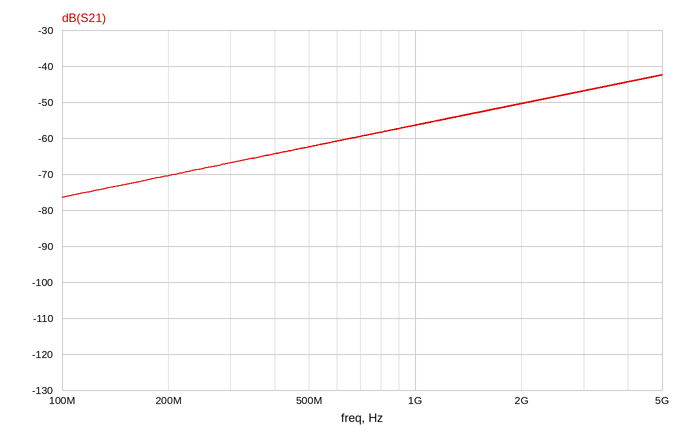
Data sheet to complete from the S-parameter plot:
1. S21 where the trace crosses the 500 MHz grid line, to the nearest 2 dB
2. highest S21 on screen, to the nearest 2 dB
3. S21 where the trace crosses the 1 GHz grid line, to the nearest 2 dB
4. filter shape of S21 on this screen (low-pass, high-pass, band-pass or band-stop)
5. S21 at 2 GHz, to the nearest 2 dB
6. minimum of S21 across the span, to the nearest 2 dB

-62 dB
-42 dB
-56 dB
high-pass
-50 dB
-76 dB
